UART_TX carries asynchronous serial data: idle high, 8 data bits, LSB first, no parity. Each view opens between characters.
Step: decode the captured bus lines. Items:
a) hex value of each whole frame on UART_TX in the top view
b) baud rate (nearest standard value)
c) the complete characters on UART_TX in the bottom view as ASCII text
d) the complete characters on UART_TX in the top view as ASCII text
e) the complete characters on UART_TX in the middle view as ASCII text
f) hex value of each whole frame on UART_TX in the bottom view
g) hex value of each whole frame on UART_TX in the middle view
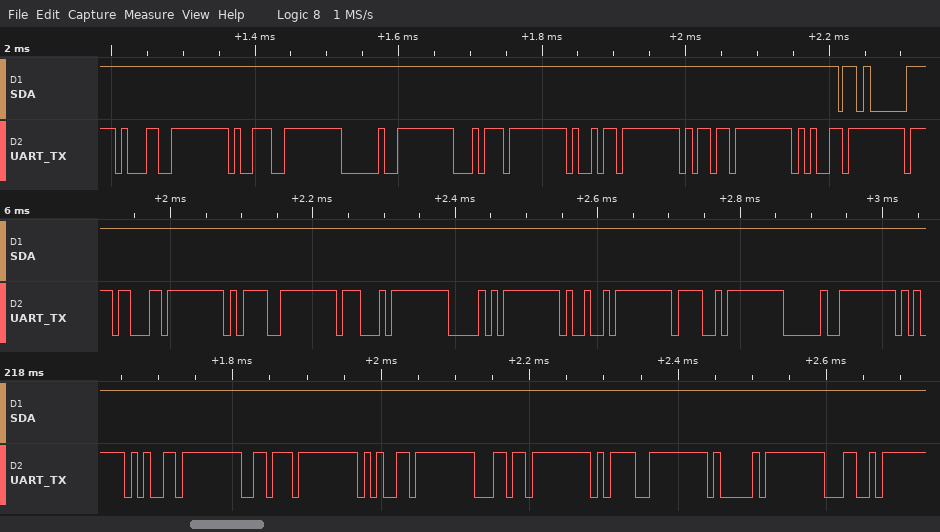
31, 39, 20, 74, 69, 6D, 65
115200 baud
"evel=AL"
"19 time"
"c=GPIO "
65, 76, 65, 6C, 3D, 41, 4C
63, 3D, 47, 50, 49, 4F, 20
